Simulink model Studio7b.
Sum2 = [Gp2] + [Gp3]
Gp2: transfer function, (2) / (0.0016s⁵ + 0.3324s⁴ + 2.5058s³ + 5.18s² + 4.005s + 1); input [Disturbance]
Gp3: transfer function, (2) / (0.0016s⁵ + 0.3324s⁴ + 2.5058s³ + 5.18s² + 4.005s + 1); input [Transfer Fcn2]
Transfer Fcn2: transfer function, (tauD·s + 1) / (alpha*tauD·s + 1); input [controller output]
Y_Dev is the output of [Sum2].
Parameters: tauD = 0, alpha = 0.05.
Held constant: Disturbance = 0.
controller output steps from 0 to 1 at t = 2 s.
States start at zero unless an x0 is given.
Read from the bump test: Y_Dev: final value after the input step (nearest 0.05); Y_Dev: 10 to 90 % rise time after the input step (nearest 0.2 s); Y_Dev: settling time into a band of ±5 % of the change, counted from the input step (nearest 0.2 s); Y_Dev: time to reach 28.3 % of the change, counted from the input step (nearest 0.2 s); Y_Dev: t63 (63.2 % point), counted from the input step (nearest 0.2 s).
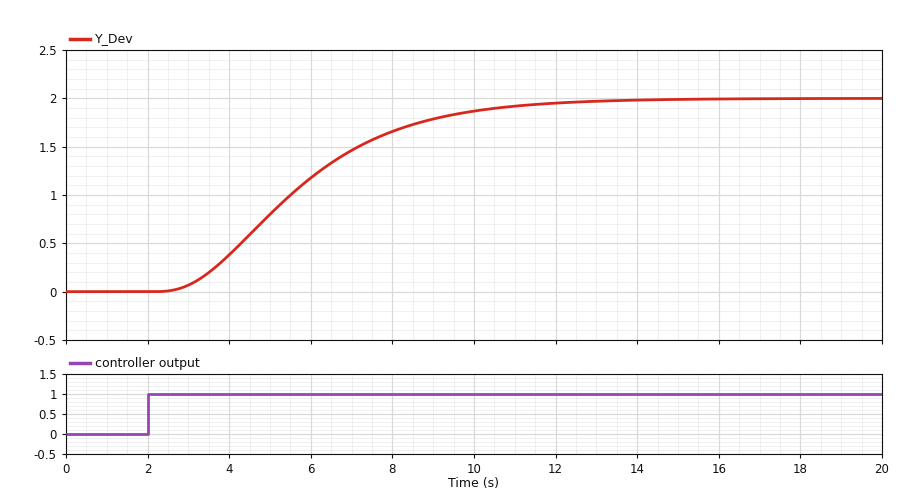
2.00
5.6 s
8.6 s
2.4 s
4.2 s
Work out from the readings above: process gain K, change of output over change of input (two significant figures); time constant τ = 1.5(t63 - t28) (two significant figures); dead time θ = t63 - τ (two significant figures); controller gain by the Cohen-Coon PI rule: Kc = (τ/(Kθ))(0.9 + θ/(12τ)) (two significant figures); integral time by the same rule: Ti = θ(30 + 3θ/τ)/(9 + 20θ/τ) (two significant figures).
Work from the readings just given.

2.0
2.7 s
1.5 s
0.85
2.4 s
